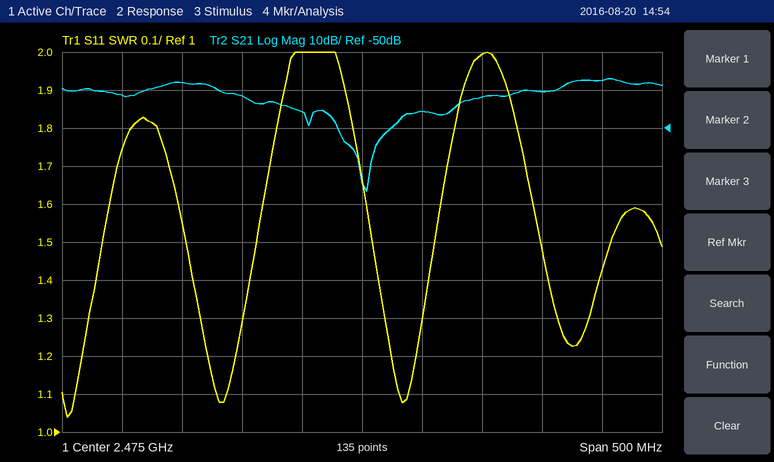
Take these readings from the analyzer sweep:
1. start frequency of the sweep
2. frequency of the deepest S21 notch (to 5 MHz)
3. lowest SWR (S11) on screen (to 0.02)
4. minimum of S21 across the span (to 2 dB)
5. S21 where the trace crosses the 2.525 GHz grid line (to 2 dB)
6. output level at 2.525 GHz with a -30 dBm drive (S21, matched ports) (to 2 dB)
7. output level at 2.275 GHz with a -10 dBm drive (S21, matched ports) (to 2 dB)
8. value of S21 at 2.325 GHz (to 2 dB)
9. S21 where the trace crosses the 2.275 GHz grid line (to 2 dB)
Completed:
2.225 GHz
2.480 GHz
1.04
-66 dB
-46 dB
-76 dBm
-52 dBm
-38 dB
-42 dB
